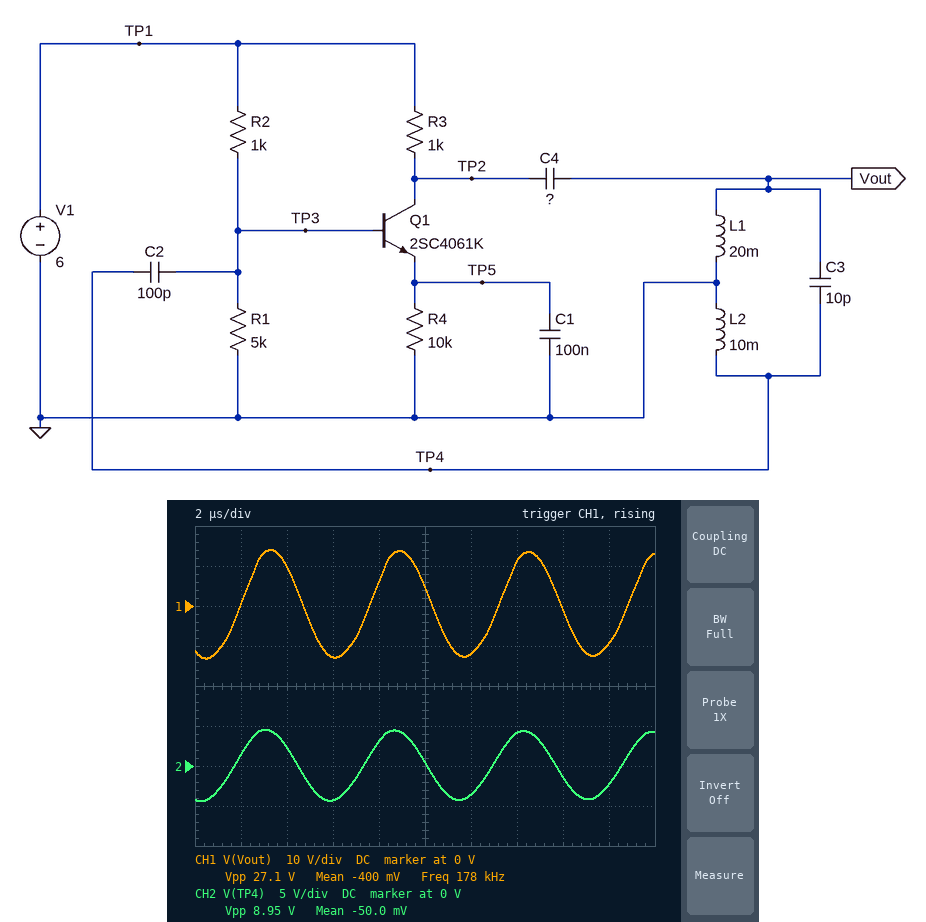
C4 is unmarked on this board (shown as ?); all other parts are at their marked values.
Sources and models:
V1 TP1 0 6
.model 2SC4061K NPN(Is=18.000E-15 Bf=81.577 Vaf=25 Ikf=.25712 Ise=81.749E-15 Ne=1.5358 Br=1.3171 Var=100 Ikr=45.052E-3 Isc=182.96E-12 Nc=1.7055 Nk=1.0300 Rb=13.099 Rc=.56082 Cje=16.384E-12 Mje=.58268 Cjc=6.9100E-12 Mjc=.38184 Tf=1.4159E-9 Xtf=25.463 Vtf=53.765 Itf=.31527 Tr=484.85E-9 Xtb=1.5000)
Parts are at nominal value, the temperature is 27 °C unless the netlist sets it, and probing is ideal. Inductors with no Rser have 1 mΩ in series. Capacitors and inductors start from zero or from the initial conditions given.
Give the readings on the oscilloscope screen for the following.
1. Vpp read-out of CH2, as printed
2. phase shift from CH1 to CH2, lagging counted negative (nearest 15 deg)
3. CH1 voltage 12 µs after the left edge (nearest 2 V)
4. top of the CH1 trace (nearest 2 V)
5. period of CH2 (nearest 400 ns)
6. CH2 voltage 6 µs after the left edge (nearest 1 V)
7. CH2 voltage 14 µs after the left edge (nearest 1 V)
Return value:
8.95 V
15 deg
-12 V
14 V
5.6 µs
-4 V
4 V
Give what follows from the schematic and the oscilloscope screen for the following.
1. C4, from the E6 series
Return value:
33 pF
